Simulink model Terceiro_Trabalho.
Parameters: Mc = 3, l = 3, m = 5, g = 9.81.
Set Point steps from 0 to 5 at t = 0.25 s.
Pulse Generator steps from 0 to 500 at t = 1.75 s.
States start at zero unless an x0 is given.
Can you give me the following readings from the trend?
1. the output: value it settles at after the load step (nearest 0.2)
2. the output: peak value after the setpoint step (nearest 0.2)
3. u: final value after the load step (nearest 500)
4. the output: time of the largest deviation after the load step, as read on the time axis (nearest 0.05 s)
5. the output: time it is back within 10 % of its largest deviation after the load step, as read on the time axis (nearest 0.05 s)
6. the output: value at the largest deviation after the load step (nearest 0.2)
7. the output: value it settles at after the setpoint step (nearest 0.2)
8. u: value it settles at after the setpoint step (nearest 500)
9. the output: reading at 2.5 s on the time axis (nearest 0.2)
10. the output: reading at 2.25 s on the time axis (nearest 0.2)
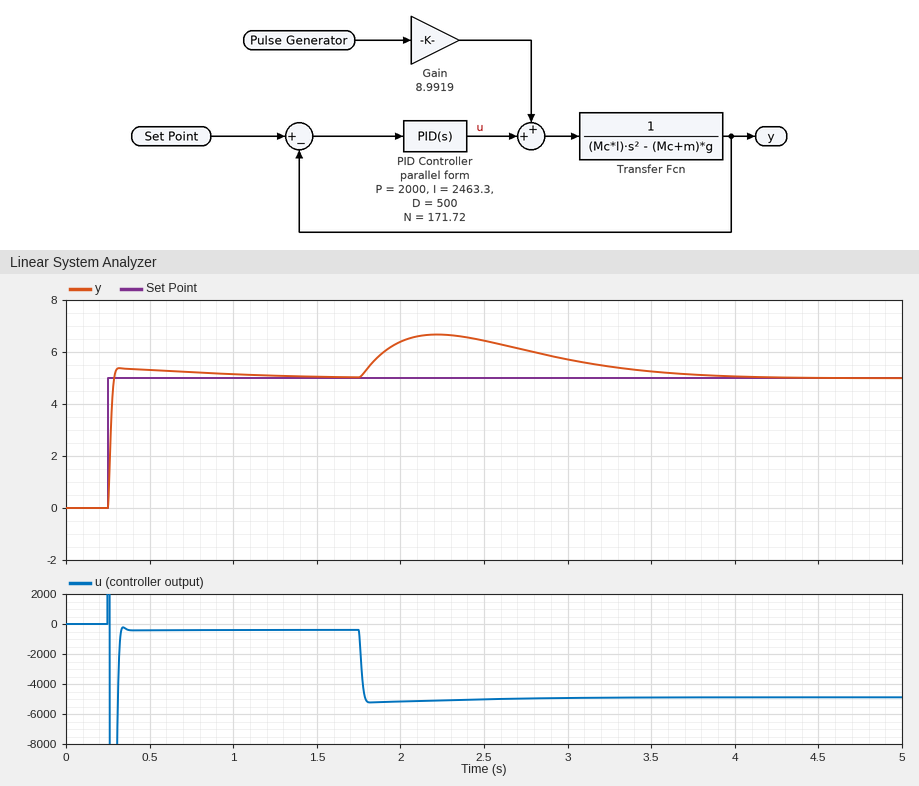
5.0
5.4
-5000
2.20 s
3.65 s
6.6
5.0
-500
6.4
6.6
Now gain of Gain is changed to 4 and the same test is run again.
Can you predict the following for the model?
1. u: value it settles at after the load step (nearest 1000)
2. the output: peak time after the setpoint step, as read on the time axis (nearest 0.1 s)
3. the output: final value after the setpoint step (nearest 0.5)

-2000
0.3 s
5.0
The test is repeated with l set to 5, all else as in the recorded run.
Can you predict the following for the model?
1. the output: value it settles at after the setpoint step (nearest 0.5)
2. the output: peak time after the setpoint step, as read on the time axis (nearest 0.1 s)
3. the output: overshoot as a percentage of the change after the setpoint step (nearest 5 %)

5.0
0.4 s
10 %
